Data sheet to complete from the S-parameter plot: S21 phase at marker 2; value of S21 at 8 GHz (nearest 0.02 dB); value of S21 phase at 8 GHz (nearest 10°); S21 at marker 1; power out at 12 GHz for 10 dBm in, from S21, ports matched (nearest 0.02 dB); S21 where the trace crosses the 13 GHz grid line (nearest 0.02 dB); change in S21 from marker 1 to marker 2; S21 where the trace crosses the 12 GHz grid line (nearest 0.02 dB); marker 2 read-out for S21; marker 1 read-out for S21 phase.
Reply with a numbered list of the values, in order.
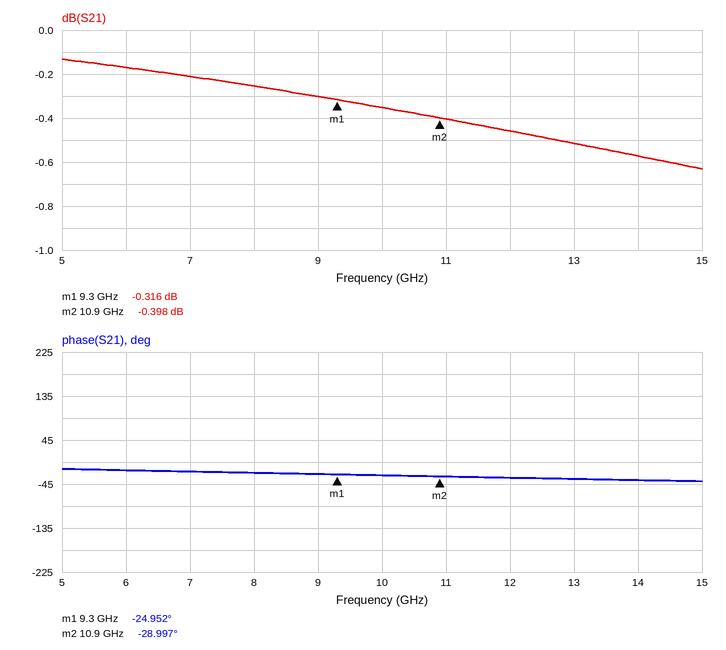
1. -28.997°
2. -0.26 dB
3. -20°
4. -0.316 dB
5. 9.54 dBm
6. -0.52 dB
7. -0.082 dB
8. -0.46 dB
9. -0.398 dB
10. -24.952°
